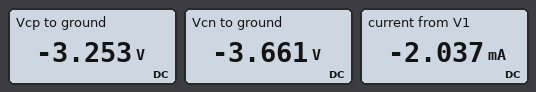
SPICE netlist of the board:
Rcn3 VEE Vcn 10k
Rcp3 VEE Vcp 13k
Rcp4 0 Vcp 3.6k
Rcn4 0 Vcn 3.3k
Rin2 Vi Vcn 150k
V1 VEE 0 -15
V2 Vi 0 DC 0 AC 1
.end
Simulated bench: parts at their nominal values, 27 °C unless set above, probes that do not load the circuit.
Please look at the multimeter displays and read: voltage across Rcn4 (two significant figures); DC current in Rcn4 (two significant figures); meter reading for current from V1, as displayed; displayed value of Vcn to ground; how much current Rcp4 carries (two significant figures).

3.7 V
1.1 mA
-2.037 mA
-3.661 V
900 µA
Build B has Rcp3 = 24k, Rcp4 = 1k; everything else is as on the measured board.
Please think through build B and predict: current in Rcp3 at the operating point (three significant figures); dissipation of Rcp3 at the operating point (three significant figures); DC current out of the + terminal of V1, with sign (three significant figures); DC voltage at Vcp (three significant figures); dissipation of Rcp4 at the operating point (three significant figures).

600 µA
8.64 mW
-1.73 mA
-600 mV
360 µW
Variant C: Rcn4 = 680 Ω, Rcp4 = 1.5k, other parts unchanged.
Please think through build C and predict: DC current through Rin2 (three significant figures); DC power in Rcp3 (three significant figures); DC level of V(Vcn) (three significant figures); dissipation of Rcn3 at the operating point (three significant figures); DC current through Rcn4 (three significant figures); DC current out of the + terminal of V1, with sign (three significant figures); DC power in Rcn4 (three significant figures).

6.34 µA
13.9 mW
-951 mV
19.7 mW
1.40 mA
-2.44 mA
1.33 mW
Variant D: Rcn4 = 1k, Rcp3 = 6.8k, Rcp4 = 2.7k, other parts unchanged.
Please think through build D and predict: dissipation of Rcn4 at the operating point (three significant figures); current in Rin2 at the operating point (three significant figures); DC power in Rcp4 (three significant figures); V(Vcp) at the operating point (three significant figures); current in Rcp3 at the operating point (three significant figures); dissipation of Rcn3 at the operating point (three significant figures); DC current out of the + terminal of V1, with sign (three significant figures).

1.84 mW
9.04 µA
6.73 mW
-4.26 V
1.58 mA
18.6 mW
-2.94 mA
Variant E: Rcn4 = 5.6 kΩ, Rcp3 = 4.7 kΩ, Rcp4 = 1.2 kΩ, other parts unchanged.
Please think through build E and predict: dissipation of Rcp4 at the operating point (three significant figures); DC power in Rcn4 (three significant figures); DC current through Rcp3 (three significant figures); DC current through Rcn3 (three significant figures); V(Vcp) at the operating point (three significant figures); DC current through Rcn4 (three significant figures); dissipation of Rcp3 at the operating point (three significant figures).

7.76 mW
4.94 mW
2.54 mA
974 µA
-3.05 V
939 µA
30.4 mW
